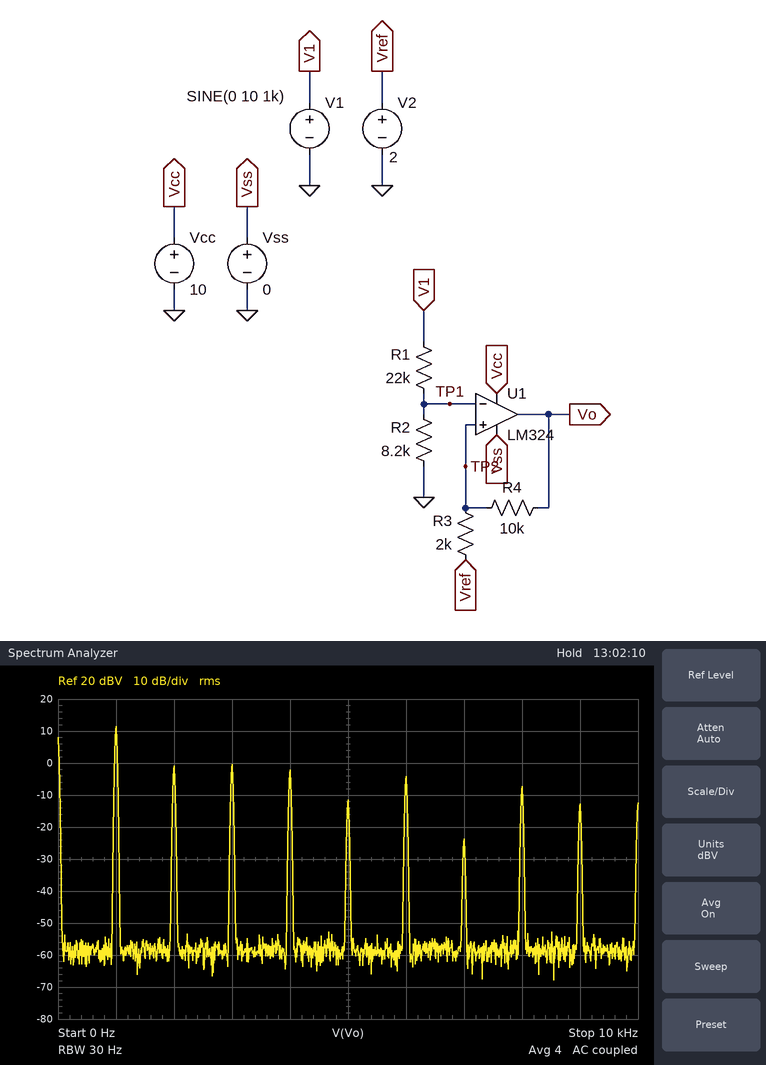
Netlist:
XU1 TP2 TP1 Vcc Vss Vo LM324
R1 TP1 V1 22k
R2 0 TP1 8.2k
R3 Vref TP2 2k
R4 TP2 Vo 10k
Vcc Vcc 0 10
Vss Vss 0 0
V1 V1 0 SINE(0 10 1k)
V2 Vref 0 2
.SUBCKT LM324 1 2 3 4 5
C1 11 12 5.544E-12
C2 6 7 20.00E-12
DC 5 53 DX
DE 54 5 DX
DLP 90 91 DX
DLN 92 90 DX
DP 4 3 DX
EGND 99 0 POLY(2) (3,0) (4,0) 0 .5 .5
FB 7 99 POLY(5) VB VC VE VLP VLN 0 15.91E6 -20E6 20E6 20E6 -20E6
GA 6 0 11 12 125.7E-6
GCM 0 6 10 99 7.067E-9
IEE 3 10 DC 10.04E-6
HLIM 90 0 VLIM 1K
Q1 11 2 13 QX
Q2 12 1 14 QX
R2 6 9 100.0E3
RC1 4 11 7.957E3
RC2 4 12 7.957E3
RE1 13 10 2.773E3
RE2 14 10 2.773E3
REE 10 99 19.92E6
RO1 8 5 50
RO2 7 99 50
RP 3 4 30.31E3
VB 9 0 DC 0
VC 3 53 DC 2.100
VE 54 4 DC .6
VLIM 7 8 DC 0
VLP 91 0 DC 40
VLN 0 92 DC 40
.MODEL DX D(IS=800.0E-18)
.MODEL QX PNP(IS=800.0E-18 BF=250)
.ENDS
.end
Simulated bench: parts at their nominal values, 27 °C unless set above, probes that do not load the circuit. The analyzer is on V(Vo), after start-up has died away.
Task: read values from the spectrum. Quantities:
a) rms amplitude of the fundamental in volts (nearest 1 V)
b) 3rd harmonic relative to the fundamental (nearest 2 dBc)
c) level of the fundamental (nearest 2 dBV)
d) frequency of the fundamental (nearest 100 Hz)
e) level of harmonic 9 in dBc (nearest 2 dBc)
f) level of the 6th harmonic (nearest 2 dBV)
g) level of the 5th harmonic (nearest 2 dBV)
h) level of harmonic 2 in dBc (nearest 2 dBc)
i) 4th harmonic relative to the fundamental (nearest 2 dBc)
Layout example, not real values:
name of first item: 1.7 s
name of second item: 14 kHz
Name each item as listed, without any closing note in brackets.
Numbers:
rms amplitude of the fundamental in volts: 4 V
3rd harmonic relative to the fundamental: -12 dBc
level of the fundamental: 12 dBV
frequency of the fundamental: 1.0 kHz
level of harmonic 9 in dBc: -24 dBc
level of the 6th harmonic: -4 dBV
level of the 5th harmonic: -12 dBV
level of harmonic 2 in dBc: -12 dBc
4th harmonic relative to the fundamental: -14 dBc
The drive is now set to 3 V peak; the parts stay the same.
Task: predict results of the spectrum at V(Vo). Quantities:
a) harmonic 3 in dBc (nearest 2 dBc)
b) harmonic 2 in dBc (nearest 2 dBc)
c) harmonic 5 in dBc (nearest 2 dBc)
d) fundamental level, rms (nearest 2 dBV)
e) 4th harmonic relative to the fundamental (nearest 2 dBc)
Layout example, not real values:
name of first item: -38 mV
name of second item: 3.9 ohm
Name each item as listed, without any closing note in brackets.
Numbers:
harmonic 3 in dBc: -6 dBc
harmonic 2 in dBc: -2 dBc
harmonic 5 in dBc: -32 dBc
fundamental level, rms: 6 dBV
4th harmonic relative to the fundamental: -12 dBc
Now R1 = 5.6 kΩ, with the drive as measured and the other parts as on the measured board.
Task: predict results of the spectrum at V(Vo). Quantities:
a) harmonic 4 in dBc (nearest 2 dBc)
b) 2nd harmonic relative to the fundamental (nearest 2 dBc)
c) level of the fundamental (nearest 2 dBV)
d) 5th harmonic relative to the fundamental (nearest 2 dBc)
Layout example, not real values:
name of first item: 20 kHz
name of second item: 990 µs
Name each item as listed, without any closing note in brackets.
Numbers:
harmonic 4 in dBc: 6 dBc
2nd harmonic relative to the fundamental: 10 dBc
level of the fundamental: -4 dBV
5th harmonic relative to the fundamental: 4 dBc
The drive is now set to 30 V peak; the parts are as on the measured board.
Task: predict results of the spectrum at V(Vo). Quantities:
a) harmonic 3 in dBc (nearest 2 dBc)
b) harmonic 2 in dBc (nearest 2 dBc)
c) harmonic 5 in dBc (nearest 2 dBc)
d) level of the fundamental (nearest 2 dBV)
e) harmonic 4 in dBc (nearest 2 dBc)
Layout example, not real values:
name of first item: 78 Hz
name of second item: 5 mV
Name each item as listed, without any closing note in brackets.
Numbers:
harmonic 3 in dBc: 2 dBc
harmonic 2 in dBc: 10 dBc
harmonic 5 in dBc: 4 dBc
level of the fundamental: -8 dBV
harmonic 4 in dBc: 8 dBc
